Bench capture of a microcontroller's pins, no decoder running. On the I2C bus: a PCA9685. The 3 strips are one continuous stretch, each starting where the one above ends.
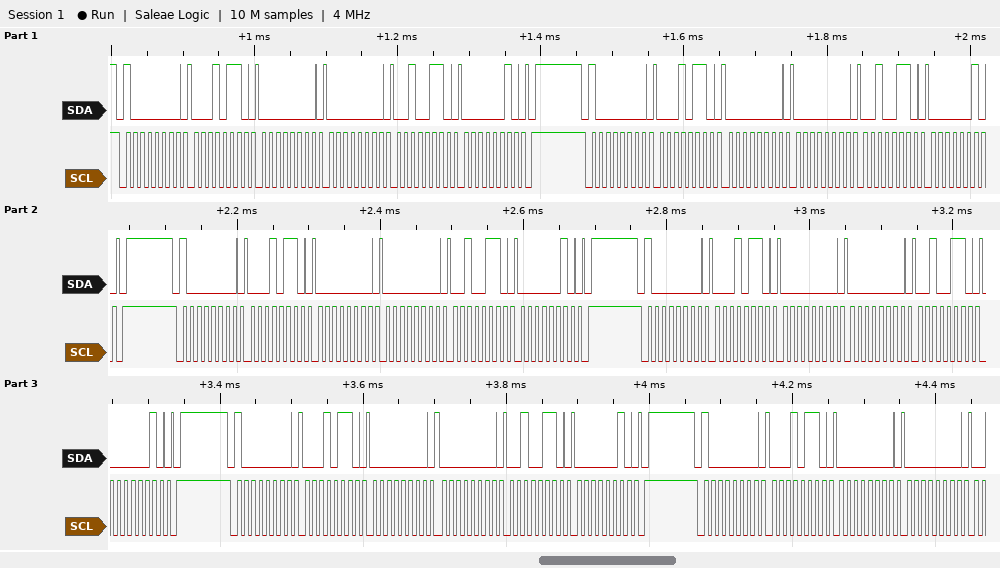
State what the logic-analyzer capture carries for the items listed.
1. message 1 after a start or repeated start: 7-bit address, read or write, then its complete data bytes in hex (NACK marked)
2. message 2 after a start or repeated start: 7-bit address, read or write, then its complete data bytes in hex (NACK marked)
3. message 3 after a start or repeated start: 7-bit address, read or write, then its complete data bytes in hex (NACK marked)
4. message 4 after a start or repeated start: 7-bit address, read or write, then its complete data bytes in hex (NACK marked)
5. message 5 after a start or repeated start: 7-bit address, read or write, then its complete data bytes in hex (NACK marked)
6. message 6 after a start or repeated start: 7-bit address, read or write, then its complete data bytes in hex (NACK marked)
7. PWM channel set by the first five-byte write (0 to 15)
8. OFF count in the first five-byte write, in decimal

0x40 write: 16 00 00 26 02
0x40 write: 16 00 00 26 02
0x40 write: 16 00 00 26 02
0x40 write: 16 00 00 26 02
0x40 write: 16 00 00 26 02
0x40 write: 16 00 00
4
550
